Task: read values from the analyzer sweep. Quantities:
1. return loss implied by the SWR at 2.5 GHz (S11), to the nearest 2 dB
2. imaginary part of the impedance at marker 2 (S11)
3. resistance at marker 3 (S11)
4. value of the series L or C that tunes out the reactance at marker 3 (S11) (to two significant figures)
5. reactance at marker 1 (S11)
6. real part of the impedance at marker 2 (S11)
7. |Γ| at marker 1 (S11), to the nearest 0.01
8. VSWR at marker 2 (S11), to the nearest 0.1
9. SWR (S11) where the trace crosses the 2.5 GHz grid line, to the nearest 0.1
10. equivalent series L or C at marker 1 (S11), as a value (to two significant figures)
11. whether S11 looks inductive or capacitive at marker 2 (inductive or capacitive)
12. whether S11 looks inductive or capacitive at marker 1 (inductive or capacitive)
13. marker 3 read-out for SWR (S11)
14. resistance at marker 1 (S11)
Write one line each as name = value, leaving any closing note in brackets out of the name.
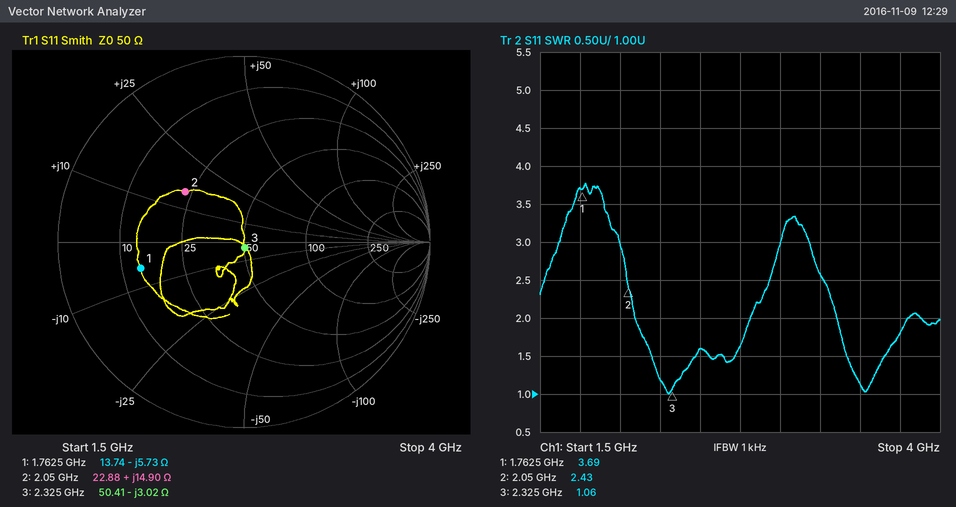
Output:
return loss implied by the SWR at 2.5 GHz (S11), to the nearest 2 dB = 12 dB
imaginary part of the impedance at marker 2 = +14.90 Ω
resistance at marker 3 = 50.41 Ω
value of the series L or C that tunes out the reactance at marker 3 (S11) = 210 pH
reactance at marker 1 = -5.73 Ω
real part of the impedance at marker 2 = 22.88 Ω
|Γ| at marker 1 (S11), to the nearest 0.01 = 0.57
VSWR at marker 2 (S11), to the nearest 0.1 = 2.4
SWR (S11) where the trace crosses the 2.5 GHz grid line, to the nearest 0.1 = 1.6
equivalent series L or C at marker 1 (S11), as a value = 16 pF
whether S11 looks inductive or capacitive at marker 2 = inductive
whether S11 looks inductive or capacitive at marker 1 = capacitive
marker 3 read-out for SWR = 1.06
resistance at marker 1 = 13.74 Ω
